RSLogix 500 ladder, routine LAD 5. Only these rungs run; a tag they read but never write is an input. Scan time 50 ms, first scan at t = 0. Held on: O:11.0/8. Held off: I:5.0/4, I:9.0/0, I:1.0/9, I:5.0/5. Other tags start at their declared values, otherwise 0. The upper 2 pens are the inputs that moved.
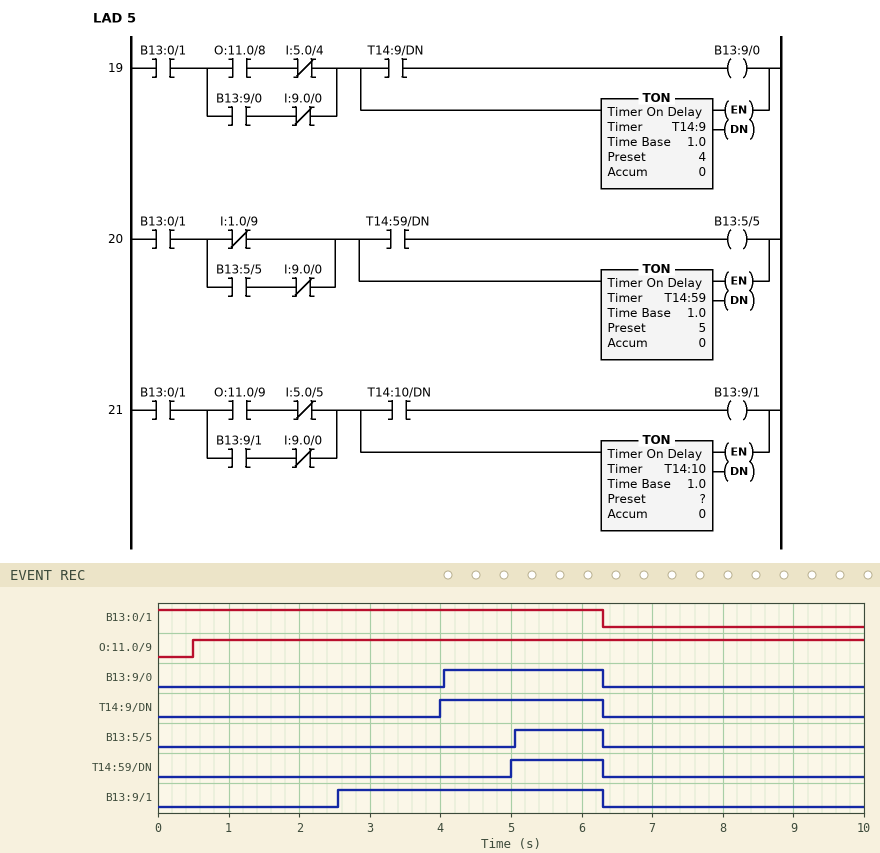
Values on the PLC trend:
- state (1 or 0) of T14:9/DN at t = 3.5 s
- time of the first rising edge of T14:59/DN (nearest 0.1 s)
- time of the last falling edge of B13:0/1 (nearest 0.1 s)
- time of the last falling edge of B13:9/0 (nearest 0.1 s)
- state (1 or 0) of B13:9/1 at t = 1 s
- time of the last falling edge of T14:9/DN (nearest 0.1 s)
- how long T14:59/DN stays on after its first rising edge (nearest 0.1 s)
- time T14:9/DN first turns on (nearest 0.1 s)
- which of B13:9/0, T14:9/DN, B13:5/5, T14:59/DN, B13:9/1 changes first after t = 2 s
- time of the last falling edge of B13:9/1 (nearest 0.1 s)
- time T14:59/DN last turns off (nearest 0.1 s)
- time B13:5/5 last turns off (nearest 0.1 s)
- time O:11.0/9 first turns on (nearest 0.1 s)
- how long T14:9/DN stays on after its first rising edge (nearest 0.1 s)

0
5.0 s
6.3 s
6.3 s
0
6.3 s
1.3 s
4.0 s
B13:9/1
6.3 s
6.3 s
6.3 s
0.5 s
2.3 s
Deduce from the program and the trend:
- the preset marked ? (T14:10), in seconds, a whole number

2 s
